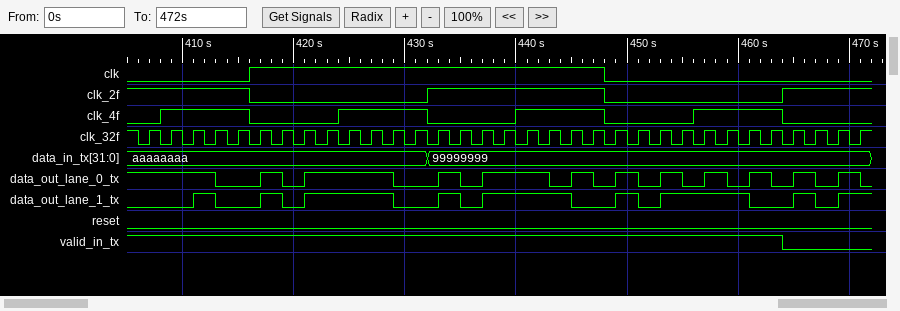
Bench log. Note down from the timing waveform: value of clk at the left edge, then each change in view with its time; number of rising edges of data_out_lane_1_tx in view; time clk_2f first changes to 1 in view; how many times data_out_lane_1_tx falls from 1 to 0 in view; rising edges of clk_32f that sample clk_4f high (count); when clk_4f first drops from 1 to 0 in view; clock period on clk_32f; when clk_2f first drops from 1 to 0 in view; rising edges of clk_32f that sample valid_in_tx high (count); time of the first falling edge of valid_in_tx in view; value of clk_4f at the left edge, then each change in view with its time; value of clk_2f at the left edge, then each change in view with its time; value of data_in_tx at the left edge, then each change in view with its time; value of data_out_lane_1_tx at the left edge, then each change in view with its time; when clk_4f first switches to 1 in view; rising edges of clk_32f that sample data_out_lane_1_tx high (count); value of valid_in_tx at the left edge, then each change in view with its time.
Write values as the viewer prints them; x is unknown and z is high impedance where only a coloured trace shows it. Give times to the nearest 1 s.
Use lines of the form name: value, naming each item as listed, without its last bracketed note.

value of clk at the left edge, then each change in view with its time: 0, 1 at 416 s, 0 at 448 s
number of rising edges of data_out_lane_1_tx in view: 9
time clk_2f first changes to 1 in view: 432 s
how many times data_out_lane_1_tx falls from 1 to 0 in view: 8
rising edges of clk_32f that sample clk_4f high: 16
when clk_4f first drops from 1 to 0 in view: 416 s
clock period on clk_32f: 2 s
when clk_2f first drops from 1 to 0 in view: 416 s
rising edges of clk_32f that sample valid_in_tx high: 29
time of the first falling edge of valid_in_tx in view: 464 s
value of clk_4f at the left edge, then each change in view with its time: 0, 1 at 408 s, 0 at 416 s, 1 at 424 s, 0 at 432 s, 1 at 440 s, 0 at 448 s, 1 at 456 s, 0 at 464 s
value of clk_2f at the left edge, then each change in view with its time: 1, 0 at 416 s, 1 at 432 s, 0 at 448 s, 1 at 464 s
value of data_in_tx at the left edge, then each change in view with its time: aaaaaaaa, 99999999 at 432 s
value of data_out_lane_1_tx at the left edge, then each change in view with its time: 0, 1 at 411 s, 0 at 413 s, 1 at 417 s, 0 at 419 s, 1 at 421 s, 0 at 429 s, 1 at 433 s, 0 at 435 s, 1 at 437 s, 0 at 445 s, 1 at 449 s, 0 at 451 s, 1 at 453 s, 0 at 461 s, 1 at 465 s, 0 at 467 s, 1 at 469 s
when clk_4f first switches to 1 in view: 408 s
rising edges of clk_32f that sample data_out_lane_1_tx high: 18
value of valid_in_tx at the left edge, then each change in view with its time: 1, 0 at 464 s
